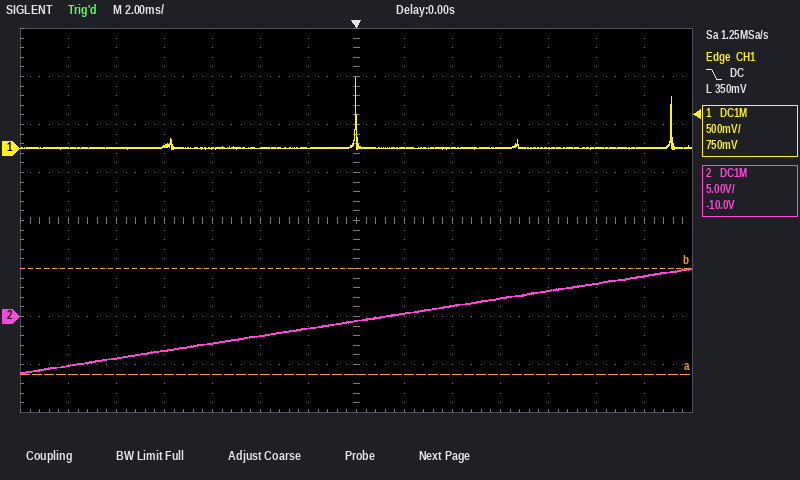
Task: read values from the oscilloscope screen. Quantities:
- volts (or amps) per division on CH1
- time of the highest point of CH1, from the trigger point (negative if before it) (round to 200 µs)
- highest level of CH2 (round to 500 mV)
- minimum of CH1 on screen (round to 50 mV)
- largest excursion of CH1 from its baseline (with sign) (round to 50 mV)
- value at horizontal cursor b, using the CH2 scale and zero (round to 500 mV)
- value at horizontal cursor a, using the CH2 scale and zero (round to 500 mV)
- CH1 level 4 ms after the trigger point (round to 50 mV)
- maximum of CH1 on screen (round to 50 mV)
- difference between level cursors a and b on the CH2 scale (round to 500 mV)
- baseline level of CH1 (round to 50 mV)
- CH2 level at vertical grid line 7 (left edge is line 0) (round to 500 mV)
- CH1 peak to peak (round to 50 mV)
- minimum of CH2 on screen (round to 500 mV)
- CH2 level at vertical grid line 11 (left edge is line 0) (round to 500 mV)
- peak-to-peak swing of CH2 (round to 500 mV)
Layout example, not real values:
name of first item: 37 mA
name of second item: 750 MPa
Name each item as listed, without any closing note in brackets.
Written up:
volts (or amps) per division on CH1: 500 mV
time of the highest point of CH1, from the trigger point (negative if before it): 0.0 ms
highest level of CH2: 5.0 V
minimum of CH1 on screen: 0 mV
largest excursion of CH1 from its baseline (with sign): +750 mV
value at horizontal cursor b, using the CH2 scale and zero: 5.0 V
value at horizontal cursor a, using the CH2 scale and zero: -6.0 V
CH1 level 4 ms after the trigger point: 0 mV
maximum of CH1 on screen: 750 mV
difference between level cursors a and b on the CH2 scale: 11.0 V
baseline level of CH1: 0 mV
CH2 level at vertical grid line 7 (left edge is line 0): -500 mV
CH1 peak to peak: 750 mV
minimum of CH2 on screen: -6.0 V
CH2 level at vertical grid line 11 (left edge is line 0): 2.5 V
peak-to-peak swing of CH2: 11.0 V
